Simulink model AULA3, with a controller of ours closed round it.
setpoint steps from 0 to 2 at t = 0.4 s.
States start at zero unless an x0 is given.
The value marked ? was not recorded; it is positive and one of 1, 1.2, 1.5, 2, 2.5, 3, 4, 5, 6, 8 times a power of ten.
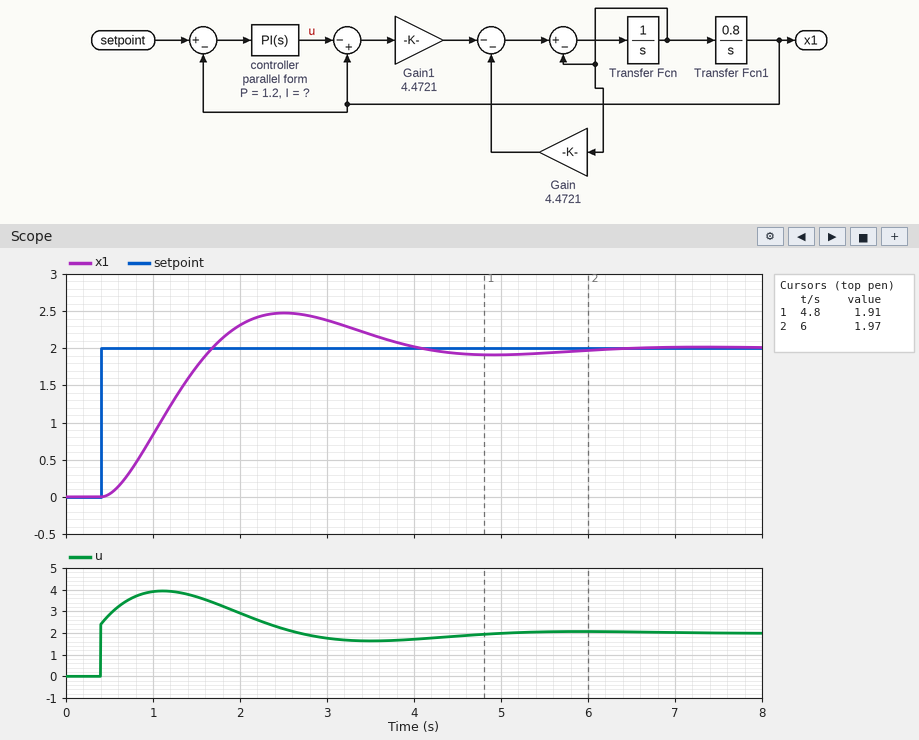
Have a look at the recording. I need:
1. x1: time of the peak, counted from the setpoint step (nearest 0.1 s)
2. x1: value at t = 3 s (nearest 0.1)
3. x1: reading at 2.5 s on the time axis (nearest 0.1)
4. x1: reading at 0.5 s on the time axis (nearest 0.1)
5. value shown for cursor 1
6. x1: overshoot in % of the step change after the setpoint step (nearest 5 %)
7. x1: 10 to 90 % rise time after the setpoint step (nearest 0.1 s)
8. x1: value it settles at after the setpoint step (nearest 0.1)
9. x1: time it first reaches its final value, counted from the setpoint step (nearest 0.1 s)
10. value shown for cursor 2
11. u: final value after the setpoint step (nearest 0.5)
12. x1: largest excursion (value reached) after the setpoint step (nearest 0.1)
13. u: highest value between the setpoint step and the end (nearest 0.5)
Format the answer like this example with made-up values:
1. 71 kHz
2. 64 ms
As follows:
1. 2.1 s
2. 2.4
3. 2.5
4. 0.0
5. 1.91
6. 25 %
7. 0.9 s
8. 2.0
9. 1.3 s
10. 1.97
11. 2.0
12. 2.5
13. 4.0
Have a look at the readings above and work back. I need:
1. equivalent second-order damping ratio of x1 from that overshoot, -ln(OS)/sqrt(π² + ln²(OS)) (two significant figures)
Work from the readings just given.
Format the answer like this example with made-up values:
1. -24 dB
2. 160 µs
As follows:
1. 0.40
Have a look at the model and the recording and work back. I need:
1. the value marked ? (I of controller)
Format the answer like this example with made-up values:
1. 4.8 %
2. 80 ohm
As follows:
1. 2.5
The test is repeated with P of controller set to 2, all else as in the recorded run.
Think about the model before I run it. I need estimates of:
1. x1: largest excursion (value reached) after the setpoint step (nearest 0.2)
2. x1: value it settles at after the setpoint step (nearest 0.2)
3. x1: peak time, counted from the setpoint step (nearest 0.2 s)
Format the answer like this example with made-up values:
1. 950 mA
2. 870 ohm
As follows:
1. 2.2
2. 2.0
3. 1.8 s
